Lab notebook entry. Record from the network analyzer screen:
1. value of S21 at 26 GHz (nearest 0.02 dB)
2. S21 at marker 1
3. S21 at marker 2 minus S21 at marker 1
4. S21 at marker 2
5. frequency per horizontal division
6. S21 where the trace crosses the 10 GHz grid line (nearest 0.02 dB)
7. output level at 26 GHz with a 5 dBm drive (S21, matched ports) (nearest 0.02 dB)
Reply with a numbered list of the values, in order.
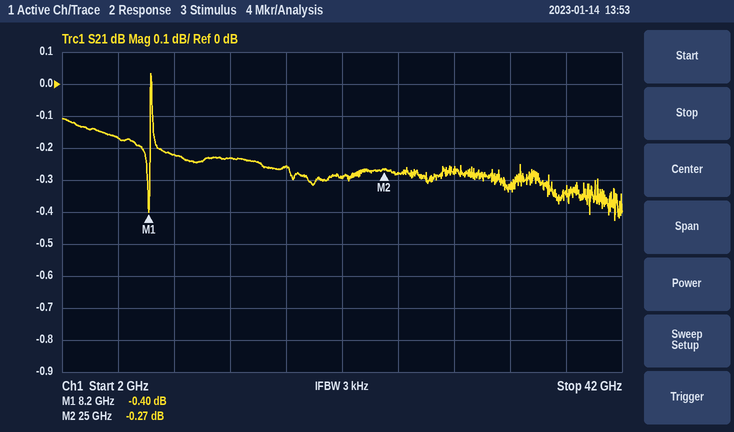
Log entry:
1. -0.28 dB
2. -0.40 dB
3. 0.13 dB
4. -0.27 dB
5. 4 GHz
6. -0.22 dB
7. 4.72 dBm
